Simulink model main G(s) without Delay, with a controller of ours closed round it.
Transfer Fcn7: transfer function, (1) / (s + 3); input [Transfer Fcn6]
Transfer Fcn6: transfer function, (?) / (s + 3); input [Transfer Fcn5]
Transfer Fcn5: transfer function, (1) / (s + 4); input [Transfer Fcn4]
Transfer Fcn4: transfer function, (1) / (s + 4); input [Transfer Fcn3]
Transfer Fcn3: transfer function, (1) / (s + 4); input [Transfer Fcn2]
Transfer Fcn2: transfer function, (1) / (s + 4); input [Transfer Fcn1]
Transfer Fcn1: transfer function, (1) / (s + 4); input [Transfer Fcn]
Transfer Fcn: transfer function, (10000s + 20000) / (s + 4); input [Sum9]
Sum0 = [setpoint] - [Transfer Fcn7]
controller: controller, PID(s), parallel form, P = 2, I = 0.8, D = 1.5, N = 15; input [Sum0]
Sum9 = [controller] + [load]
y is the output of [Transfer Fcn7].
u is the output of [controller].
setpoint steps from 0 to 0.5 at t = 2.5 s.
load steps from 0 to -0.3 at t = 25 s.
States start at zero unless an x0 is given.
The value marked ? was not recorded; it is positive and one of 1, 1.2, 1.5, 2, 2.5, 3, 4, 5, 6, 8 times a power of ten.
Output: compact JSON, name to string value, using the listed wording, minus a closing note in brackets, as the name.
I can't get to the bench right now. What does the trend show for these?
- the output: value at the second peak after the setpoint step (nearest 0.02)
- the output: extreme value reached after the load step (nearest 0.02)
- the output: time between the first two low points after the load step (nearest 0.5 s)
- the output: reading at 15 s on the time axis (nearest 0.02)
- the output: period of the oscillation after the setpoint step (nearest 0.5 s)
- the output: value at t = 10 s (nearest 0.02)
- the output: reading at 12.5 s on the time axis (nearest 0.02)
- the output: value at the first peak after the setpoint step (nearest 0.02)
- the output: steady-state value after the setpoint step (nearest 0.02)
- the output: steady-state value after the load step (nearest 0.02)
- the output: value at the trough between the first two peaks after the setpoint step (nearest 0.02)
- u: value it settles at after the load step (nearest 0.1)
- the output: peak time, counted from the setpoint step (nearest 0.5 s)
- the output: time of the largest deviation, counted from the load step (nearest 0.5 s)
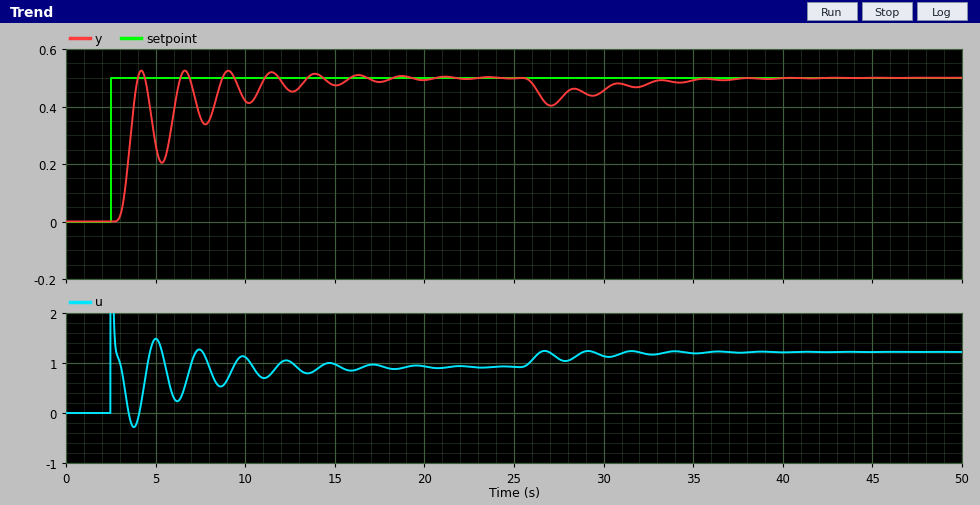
{"the output: value at the second peak after the setpoint step": "0.52", "the output: extreme value reached after the load step": "0.40", "the output: time between the first two low points after the load step": "2.5 s", "the output: reading at 15 s on the time axis": "0.48", "the output: period of the oscillation after the setpoint step": "2.5 s", "the output: value at t = 10 s": "0.42", "the output: reading at 12.5 s on the time axis": "0.46", "the output: value at the first peak after the setpoint step": "0.52", "the output: steady-state value after the setpoint step": "0.50", "the output: steady-state value after the load step": "0.50", "the output: value at the trough between the first two peaks after the setpoint step": "0.20", "u: value it settles at after the load step": "1.2", "the output: peak time, counted from the setpoint step": "1.5 s", "the output: time of the largest deviation, counted from the load step": "2.0 s"}
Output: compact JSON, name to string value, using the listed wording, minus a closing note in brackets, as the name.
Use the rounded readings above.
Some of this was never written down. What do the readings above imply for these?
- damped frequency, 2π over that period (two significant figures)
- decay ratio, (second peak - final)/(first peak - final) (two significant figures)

{"damped frequency, 2π over that period": "2.5 rad/s", "decay ratio, (second peak - final)/(first peak - final)": "1.0"}
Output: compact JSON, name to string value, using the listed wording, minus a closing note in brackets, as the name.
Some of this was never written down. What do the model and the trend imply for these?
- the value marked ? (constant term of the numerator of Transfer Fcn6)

{"the value marked ?": "1"}
